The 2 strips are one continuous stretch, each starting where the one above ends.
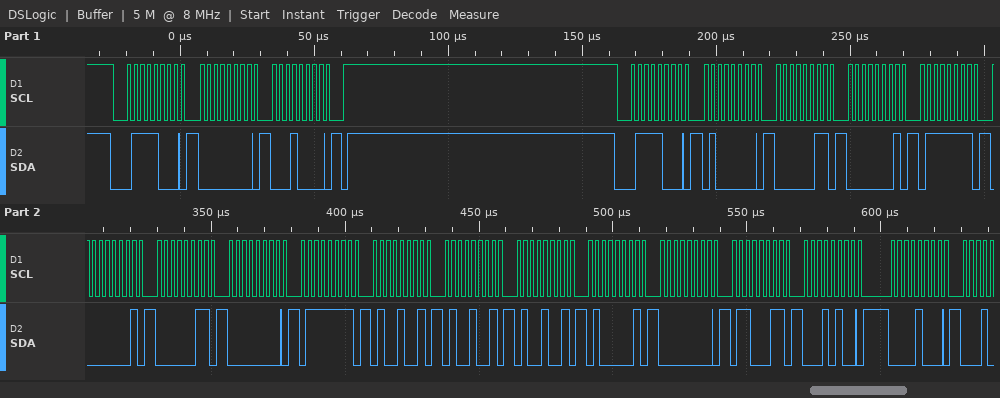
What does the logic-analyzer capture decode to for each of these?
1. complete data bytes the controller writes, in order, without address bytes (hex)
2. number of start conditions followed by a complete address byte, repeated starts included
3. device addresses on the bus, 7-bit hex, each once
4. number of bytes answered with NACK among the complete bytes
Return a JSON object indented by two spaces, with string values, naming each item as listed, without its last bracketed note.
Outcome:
{
  "complete data bytes the controller writes, in order, without address bytes": "00 10 40 03 01 7F 01 03 00 7F 49 49 49 41 00 63 14 08",
  "number of start conditions followed by a complete address byte, repeated starts included": "2",
  "device addresses on the bus, 7-bit hex, each once": "0x3C",
  "number of bytes answered with NACK among the complete bytes": "0"
}
